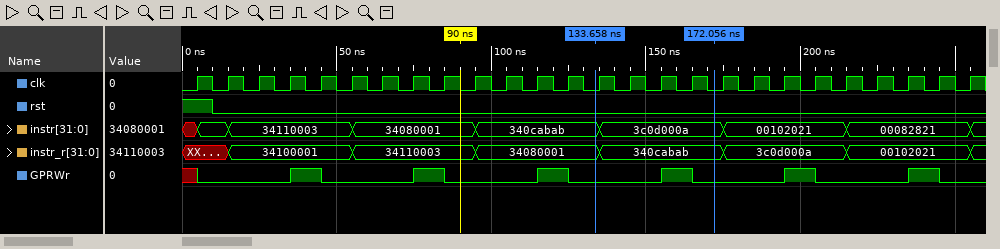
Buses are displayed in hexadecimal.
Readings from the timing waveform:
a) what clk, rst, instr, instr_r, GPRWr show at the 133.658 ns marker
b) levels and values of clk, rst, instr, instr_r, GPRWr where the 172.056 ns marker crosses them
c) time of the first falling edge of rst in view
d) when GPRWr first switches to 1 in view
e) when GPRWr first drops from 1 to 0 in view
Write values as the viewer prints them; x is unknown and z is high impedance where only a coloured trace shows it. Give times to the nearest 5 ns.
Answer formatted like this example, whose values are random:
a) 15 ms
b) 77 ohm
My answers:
a) clk=0, rst=0, instr=340cabab, instr_r=34080001, GPRWr=0
b) clk=0, rst=0, instr=3c0d000a, instr_r=340cabab, GPRWr=0
c) 10 ns
d) 35 ns
e) 45 ns
